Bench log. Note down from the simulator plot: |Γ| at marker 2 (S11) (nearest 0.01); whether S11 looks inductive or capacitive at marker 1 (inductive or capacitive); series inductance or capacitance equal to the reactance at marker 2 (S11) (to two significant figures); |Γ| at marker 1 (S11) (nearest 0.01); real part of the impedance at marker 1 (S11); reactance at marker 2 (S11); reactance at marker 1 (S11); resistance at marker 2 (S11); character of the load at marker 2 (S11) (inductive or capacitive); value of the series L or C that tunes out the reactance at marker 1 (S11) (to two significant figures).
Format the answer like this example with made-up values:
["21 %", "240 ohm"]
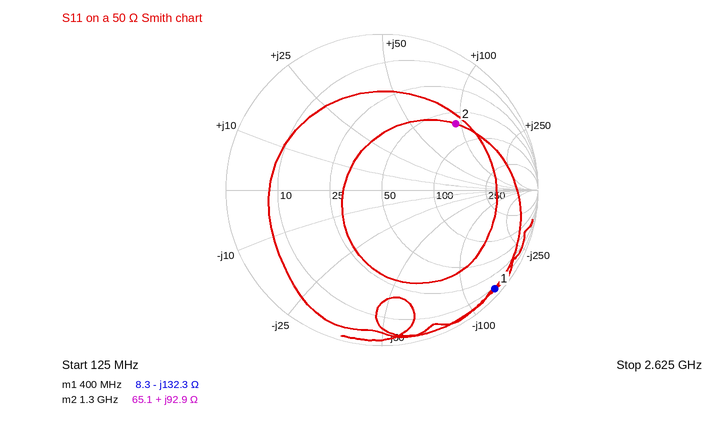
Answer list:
["0.64", "capacitive", "11 nH", "0.96", "8.3 Ω", "+92.9 Ω", "-132.3 Ω", "65.1 Ω", "inductive", "53 nH"]
